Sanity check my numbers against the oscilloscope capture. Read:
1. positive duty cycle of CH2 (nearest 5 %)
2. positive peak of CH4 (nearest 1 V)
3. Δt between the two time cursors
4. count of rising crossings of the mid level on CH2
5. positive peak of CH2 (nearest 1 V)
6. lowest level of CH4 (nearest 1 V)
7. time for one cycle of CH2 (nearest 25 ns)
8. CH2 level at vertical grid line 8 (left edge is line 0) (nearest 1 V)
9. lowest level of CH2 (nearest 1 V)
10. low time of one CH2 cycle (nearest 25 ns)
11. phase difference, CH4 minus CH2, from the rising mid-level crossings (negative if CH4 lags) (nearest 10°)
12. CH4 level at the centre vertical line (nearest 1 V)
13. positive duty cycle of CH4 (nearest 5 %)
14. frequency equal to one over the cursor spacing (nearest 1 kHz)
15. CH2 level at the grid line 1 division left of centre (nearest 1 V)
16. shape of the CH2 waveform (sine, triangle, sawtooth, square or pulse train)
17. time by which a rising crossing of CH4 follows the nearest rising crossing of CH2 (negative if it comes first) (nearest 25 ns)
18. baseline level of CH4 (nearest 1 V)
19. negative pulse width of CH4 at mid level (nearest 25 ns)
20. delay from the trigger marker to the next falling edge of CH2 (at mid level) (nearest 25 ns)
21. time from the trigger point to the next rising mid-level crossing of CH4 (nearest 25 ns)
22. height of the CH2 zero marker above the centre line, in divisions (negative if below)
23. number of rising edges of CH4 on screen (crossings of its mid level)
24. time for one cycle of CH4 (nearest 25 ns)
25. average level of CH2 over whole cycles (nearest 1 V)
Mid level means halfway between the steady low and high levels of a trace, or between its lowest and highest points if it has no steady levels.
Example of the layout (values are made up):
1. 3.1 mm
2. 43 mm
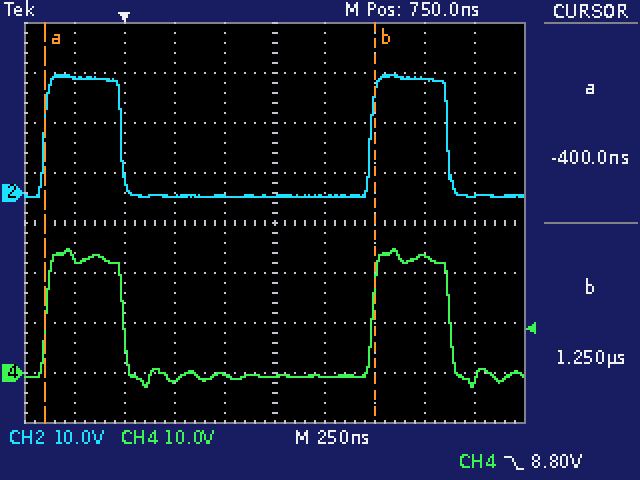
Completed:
1. 25 %
2. 25 V
3. 1.650 µs
4. 2
5. 24 V
6. -3 V
7. 1.625 µs
8. 23 V
9. -1 V
10. 1.250 µs
11. 0°
12. -1 V
13. 25 %
14. 606 kHz
15. -1 V
16. pulse train
17. 0 ns
18. -1 V
19. 1.250 µs
20. 1.625 µs
21. 1.250 µs
22. +0.6 div
23. 2
24. 1.625 µs
25. 5 V
